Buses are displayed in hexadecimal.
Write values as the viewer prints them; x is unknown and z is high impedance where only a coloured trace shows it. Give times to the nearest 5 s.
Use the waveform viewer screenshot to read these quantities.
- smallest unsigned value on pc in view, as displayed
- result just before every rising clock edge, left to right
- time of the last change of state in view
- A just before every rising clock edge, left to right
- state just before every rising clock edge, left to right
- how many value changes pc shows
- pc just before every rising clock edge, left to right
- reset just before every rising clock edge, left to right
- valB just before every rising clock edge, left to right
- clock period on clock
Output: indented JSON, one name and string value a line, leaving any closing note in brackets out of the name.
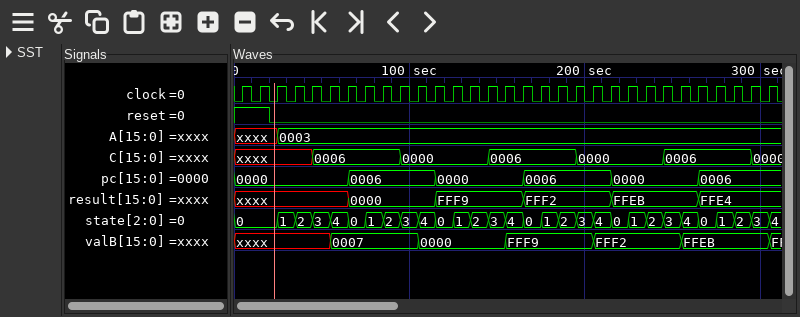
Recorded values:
{
  "smallest unsigned value on pc in view, as displayed": "0000",
  "result just before every rising clock edge, left to right": "xxxx, xxxx, xxxx, xxxx, xxxx, xxxx, xxxx, 0000, 0000, 0000, 0000, 0000, FFF9, FFF9, FFF9, FFF9, FFF9, FFF2, FFF2, FFF2, FFF2, FFF2, FFEB, FFEB, FFEB, FFEB, FFEB, FFE4, FFE4, FFE4, FFE4",
  "time of the last change of state in view": "305 s",
  "A just before every rising clock edge, left to right": "xxxx, xxxx, xxxx, 0003, 0003, 0003, 0003, 0003, 0003, 0003, 0003, 0003, 0003, 0003, 0003, 0003, 0003, 0003, 0003, 0003, 0003, 0003, 0003, 0003, 0003, 0003, 0003, 0003, 0003, 0003, 0003",
  "state just before every rising clock edge, left to right": "0, 0, 0, 1, 2, 3, 4, 0, 1, 2, 3, 4, 0, 1, 2, 3, 4, 0, 1, 2, 3, 4, 0, 1, 2, 3, 4, 0, 1, 2, 3",
  "how many value changes pc shows": "5",
  "pc just before every rising clock edge, left to right": "0000, 0000, 0000, 0000, 0000, 0000, 0000, 0006, 0006, 0006, 0006, 0006, 0000, 0000, 0000, 0000, 0000, 0006, 0006, 0006, 0006, 0006, 0000, 0000, 0000, 0000, 0000, 0006, 0006, 0006, 0006",
  "reset just before every rising clock edge, left to right": "1 1 0 0 0 0 0 0 0 0 0 0 0 0 0 0 0 0 0 0 0 0 0 0 0 0 0 0 0 0 0",
  "valB just before every rising clock edge, left to right": "xxxx, xxxx, xxxx, xxxx, xxxx, xxxx, 0007, 0007, 0007, 0007, 0007, 0000, 0000, 0000, 0000, 0000, FFF9, FFF9, FFF9, FFF9, FFF9, FFF2, FFF2, FFF2, FFF2, FFF2, FFEB, FFEB, FFEB, FFEB, FFEB",
  "clock period on clock": "10 s"
}
